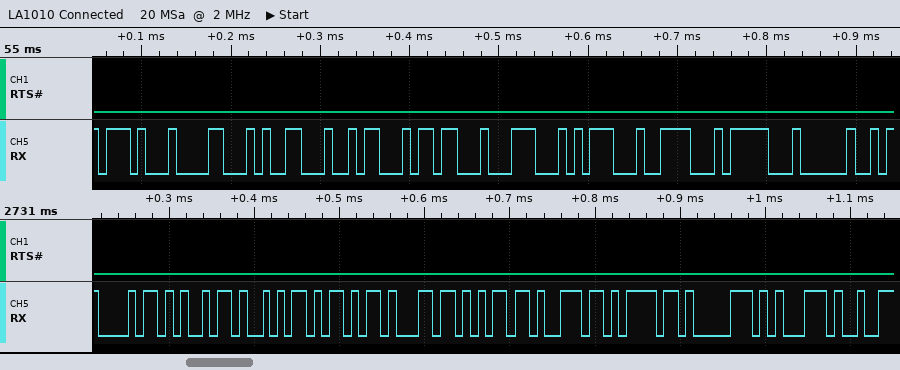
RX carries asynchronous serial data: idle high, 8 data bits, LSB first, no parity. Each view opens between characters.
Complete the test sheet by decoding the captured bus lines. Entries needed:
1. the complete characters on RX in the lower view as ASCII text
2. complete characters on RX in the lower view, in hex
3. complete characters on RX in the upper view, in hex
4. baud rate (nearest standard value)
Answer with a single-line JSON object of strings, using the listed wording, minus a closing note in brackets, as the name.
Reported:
{"the complete characters on RX in the lower view as ASCII text": "\"hijklmnopq\"", "complete characters on RX in the lower view, in hex": "68, 69, 6A, 6B, 6C, 6D, 6E, 6F, 70, 71", "complete characters on RX in the upper view, in hex": "17, 18, 19, 1A, 1B, 1C, 1D, 1E, 1F, 20", "baud rate": "115200 baud"}
